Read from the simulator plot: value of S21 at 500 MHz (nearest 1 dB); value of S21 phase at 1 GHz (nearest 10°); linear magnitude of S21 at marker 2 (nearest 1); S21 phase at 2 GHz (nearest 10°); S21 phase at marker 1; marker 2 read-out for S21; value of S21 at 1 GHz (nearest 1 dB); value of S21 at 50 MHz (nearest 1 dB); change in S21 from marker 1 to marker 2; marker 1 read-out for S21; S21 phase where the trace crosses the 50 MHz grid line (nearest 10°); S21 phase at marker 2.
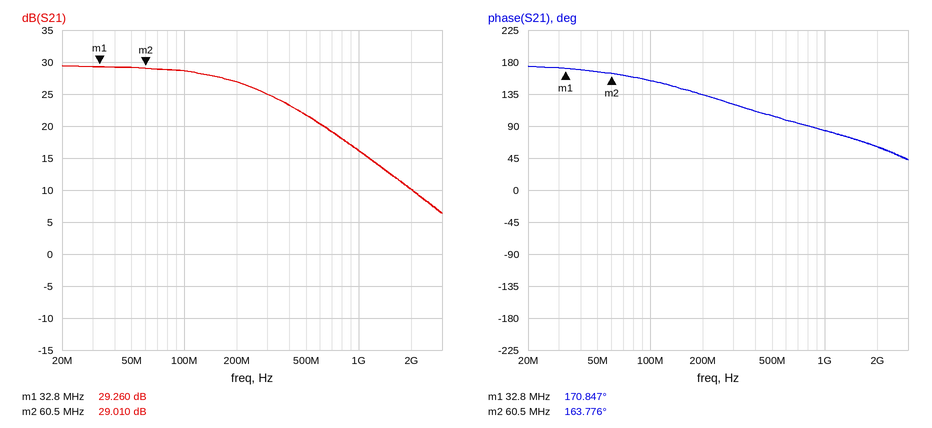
22 dB
80°
28
60°
170.847°
29.010 dB
16 dB
29 dB
-0.250 dB
29.260 dB
170°
163.776°
